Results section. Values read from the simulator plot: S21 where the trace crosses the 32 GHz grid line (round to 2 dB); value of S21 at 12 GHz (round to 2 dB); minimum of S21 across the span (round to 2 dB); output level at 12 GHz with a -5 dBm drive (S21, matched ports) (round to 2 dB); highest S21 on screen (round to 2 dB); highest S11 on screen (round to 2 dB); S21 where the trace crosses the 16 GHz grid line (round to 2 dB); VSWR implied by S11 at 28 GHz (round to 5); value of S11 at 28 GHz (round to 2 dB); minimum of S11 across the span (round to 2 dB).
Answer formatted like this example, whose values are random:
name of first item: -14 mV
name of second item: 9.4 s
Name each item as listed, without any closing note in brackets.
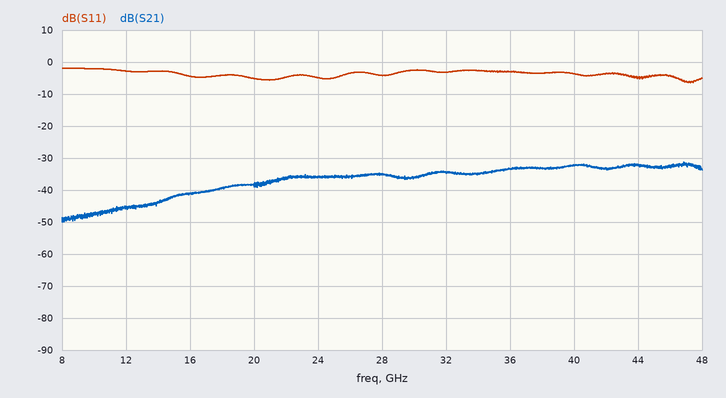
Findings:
S21 where the trace crosses the 32 GHz grid line: -34 dB
value of S21 at 12 GHz: -46 dB
minimum of S21 across the span: -50 dB
output level at 12 GHz with a -5 dBm drive (S21, matched ports): -50 dBm
highest S21 on screen: -32 dB
highest S11 on screen: -2 dB
S21 where the trace crosses the 16 GHz grid line: -42 dB
VSWR implied by S11 at 28 GHz: 5
value of S11 at 28 GHz: -4 dB
minimum of S11 across the span: -6 dB
